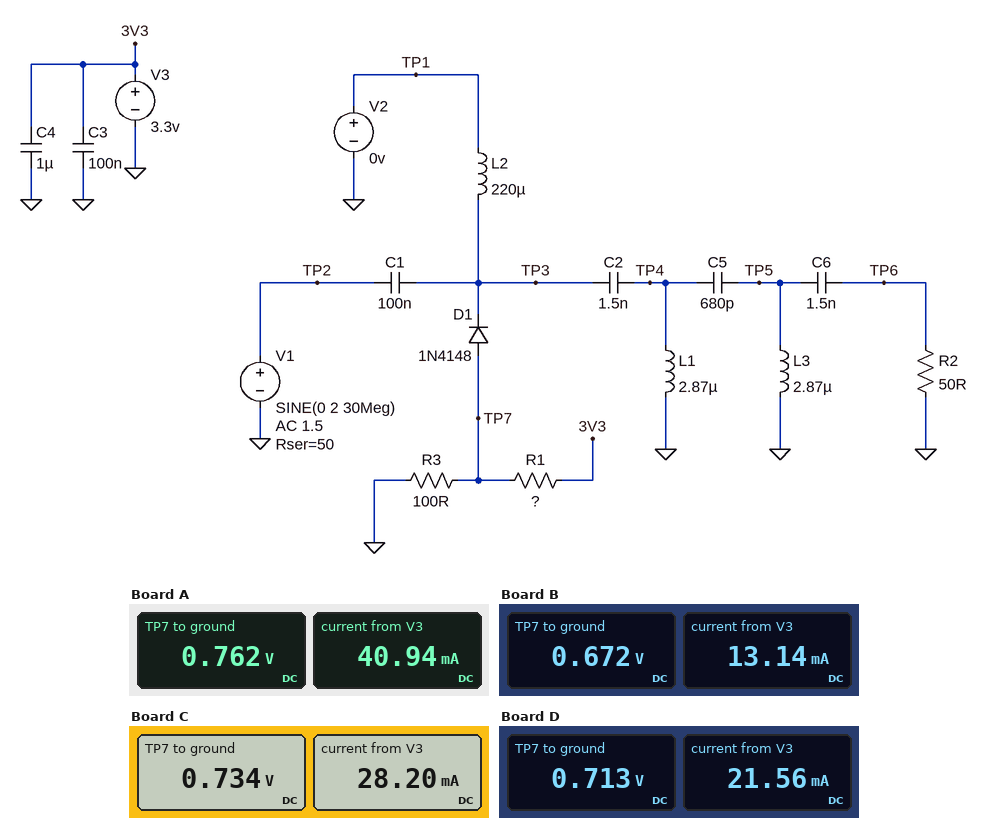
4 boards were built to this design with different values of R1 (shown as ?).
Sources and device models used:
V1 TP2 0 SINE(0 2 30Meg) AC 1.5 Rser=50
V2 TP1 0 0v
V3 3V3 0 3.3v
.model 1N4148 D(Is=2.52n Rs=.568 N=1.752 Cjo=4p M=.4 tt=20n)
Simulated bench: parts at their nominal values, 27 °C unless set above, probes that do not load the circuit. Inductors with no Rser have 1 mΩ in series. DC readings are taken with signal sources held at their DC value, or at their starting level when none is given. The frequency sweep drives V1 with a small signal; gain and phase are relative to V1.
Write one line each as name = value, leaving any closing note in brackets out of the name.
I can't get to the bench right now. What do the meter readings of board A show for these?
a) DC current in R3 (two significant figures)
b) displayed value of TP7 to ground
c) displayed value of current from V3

DC current in R3 = 7.6 mA
displayed value of TP7 to ground = 0.762 V
displayed value of current from V3 = 40.94 mA
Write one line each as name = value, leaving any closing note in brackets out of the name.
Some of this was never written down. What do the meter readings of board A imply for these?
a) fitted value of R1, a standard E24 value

fitted value of R1, a standard E24 value = 62 Ω
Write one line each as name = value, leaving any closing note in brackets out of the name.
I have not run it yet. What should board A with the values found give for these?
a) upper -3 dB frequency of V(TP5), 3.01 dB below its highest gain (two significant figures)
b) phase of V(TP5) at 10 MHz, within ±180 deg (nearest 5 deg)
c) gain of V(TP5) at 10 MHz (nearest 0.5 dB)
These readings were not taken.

upper -3 dB frequency of V(TP5), 3.01 dB below its highest gain = 3.8 MHz
phase of V(TP5) at 10 MHz, within ±180 deg = 30 deg
gain of V(TP5) at 10 MHz = -10.5 dB
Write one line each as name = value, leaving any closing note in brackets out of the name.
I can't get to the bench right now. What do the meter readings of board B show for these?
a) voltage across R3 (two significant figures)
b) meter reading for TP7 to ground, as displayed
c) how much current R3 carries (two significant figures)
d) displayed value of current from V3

voltage across R3 = 670 mV
meter reading for TP7 to ground, as displayed = 0.672 V
how much current R3 carries = 6.7 mA
displayed value of current from V3 = 13.14 mA
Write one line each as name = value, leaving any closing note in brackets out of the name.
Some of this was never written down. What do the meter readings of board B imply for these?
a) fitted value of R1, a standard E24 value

fitted value of R1, a standard E24 value = 200 Ω
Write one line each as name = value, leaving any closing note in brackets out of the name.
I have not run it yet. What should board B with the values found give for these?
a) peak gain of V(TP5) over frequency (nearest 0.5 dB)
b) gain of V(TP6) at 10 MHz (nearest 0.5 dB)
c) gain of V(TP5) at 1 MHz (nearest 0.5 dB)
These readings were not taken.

peak gain of V(TP5) over frequency = -5.5 dB
gain of V(TP6) at 10 MHz = -9.0 dB
gain of V(TP5) at 1 MHz = -38.0 dB
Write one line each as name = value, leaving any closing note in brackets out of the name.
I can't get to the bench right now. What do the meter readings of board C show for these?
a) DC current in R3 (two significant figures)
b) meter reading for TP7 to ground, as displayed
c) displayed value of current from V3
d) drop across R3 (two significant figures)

DC current in R3 = 7.3 mA
meter reading for TP7 to ground, as displayed = 0.734 V
displayed value of current from V3 = 28.20 mA
drop across R3 = 730 mV
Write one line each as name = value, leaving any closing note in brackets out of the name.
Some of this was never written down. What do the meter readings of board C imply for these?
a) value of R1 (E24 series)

value of R1 = 91 Ω
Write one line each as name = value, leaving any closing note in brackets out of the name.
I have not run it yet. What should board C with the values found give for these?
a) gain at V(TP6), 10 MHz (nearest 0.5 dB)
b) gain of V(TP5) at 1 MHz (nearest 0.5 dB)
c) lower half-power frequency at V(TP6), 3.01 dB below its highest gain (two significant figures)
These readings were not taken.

gain at V(TP6), 10 MHz = -10.0 dB
gain of V(TP5) at 1 MHz = -39.5 dB
lower half-power frequency at V(TP6), 3.01 dB below its highest gain = 1.8 MHz
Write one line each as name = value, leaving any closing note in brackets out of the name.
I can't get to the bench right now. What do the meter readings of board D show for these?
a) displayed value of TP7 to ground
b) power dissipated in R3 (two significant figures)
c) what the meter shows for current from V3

displayed value of TP7 to ground = 0.713 V
power dissipated in R3 = 5.1 mW
what the meter shows for current from V3 = 21.56 mA
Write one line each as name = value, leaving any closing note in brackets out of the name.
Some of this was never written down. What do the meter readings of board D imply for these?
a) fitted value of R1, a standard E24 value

fitted value of R1, a standard E24 value = 120 Ω
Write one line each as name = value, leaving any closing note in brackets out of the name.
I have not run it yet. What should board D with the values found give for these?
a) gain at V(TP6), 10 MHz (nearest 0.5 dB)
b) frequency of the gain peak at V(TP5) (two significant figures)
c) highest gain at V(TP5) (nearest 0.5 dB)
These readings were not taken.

gain at V(TP6), 10 MHz = -9.5 dB
frequency of the gain peak at V(TP5) = 2.0 MHz
highest gain at V(TP5) = -6.0 dB
